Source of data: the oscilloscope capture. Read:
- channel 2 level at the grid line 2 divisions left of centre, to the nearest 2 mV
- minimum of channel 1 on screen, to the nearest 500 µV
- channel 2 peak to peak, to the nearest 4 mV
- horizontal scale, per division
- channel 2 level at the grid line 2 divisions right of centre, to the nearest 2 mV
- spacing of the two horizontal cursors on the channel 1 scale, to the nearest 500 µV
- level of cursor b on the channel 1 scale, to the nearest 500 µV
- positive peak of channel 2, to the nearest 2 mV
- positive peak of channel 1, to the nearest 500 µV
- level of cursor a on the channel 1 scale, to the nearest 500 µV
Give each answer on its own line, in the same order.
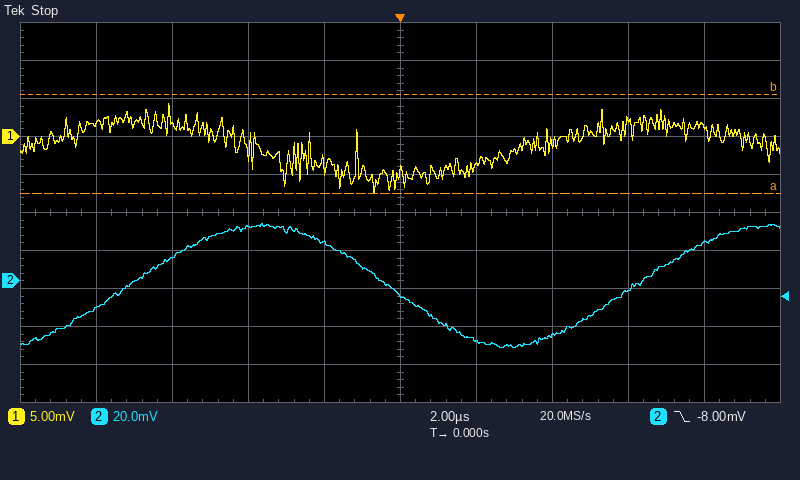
28 mV
-7.5 mV
64 mV
2 µs
-28 mV
13.0 mV
5.5 mV
30 mV
4.5 mV
-7.5 mV
